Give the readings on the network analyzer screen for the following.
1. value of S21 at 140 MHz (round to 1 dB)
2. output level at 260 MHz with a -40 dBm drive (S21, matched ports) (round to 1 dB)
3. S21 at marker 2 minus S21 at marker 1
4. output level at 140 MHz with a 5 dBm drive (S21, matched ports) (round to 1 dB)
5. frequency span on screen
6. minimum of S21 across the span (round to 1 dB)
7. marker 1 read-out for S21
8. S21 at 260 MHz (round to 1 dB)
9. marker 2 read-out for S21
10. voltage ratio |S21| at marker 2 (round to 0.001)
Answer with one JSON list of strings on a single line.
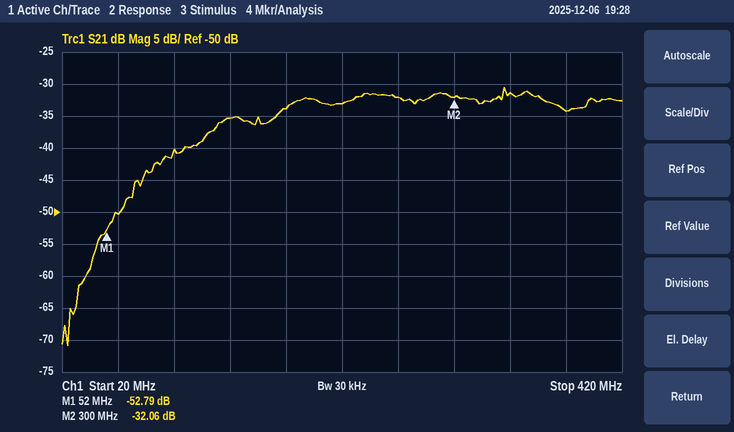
["-35 dB", "-72 dBm", "20.73 dB", "-30 dBm", "400 MHz", "-71 dB", "-52.79 dB", "-32 dB", "-32.06 dB", "0.025"]
